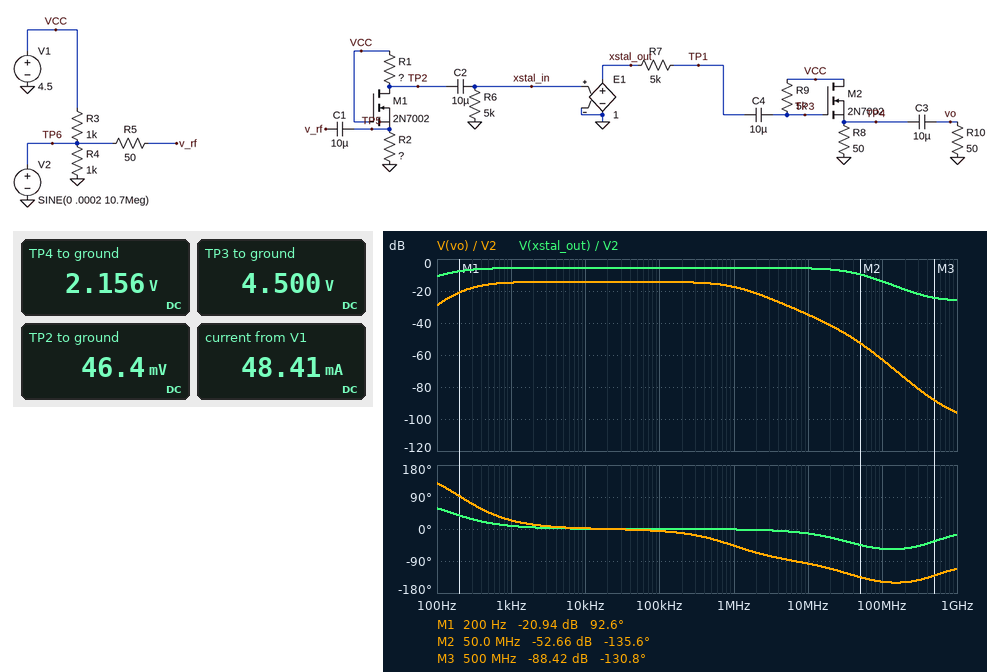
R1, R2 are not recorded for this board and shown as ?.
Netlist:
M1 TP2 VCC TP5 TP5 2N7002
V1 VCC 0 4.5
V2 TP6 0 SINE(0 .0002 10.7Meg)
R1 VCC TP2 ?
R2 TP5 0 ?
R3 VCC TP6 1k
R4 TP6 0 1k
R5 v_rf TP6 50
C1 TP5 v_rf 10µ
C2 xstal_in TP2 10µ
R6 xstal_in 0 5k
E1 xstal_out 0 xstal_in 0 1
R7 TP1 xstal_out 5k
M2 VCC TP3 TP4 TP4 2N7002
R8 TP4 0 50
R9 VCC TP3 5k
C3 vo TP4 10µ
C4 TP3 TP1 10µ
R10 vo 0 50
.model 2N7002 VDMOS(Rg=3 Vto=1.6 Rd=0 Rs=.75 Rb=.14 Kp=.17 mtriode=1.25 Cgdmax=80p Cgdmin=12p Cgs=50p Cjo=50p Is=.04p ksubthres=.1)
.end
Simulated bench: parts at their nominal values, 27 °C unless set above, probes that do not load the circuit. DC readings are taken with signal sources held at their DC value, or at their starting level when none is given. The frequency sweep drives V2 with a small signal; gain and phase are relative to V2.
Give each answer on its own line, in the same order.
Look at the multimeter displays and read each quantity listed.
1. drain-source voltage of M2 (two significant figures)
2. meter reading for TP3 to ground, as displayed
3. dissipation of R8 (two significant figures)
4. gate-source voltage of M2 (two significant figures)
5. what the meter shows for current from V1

2.3 V
4.500 V
93 mW
2.3 V
48.41 mA
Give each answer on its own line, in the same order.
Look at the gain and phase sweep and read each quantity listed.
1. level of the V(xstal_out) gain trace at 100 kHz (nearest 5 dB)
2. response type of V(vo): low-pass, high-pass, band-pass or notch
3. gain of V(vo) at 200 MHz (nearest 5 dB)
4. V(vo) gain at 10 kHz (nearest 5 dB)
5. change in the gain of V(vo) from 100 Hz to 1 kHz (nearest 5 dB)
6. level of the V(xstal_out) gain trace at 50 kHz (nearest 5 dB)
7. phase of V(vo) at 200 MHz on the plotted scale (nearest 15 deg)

-5 dB
band-pass
-75 dB
-15 dB
15 dB
-5 dB
-150 deg
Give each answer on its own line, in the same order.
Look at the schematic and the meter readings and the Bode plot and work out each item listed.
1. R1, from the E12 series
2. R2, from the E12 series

5.6 kΩ
56 Ω
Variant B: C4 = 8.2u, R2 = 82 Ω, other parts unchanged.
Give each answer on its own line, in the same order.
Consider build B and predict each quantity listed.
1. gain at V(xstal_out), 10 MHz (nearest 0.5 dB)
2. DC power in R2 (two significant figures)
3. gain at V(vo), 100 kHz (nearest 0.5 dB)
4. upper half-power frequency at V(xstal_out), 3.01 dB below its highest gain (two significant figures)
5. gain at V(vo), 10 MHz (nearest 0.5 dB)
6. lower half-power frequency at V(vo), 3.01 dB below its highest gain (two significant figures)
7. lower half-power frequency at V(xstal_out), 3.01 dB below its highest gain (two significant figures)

-4.5 dB
51 µW
-13.0 dB
35 MHz
-33.5 dB
320 Hz
120 Hz
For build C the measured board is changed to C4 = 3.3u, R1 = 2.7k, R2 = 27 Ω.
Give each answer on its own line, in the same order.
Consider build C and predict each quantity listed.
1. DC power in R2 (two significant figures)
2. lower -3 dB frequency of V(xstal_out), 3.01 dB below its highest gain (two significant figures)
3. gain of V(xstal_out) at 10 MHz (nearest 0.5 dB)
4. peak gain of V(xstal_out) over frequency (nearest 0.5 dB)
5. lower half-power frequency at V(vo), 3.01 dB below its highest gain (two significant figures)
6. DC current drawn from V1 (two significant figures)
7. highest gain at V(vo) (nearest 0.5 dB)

73 µW
210 Hz
-9.5 dB
-9.0 dB
380 Hz
49 mA
-18.0 dB
